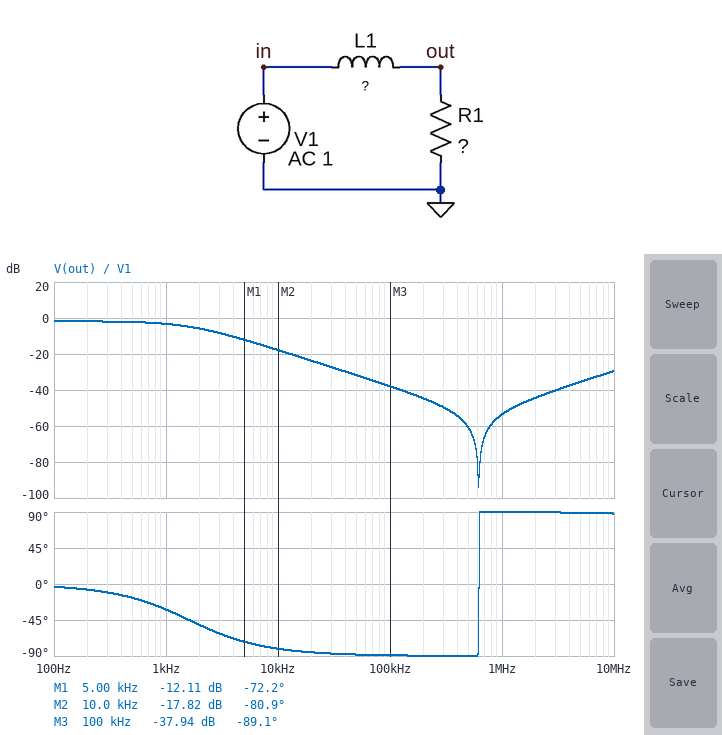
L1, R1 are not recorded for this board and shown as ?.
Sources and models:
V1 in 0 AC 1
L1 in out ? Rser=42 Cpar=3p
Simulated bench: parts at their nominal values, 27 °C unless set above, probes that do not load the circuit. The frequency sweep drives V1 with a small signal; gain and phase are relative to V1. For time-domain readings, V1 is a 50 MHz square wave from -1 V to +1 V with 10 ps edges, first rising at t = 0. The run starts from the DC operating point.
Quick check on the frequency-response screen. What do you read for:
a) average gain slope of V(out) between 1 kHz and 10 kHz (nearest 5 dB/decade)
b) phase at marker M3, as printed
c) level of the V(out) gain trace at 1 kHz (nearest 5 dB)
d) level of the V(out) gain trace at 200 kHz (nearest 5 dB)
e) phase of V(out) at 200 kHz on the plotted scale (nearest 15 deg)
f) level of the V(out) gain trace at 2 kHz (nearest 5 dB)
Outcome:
-15 dB/decade
-89.1 deg
-5 dB
-45 dB
-90 deg
-5 dB
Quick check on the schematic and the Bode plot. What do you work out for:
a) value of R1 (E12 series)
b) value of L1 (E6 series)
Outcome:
180 Ω
22 mH
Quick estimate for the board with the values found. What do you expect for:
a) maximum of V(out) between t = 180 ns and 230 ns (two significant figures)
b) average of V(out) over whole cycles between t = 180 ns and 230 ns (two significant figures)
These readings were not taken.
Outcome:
1.2 V
-810 mV
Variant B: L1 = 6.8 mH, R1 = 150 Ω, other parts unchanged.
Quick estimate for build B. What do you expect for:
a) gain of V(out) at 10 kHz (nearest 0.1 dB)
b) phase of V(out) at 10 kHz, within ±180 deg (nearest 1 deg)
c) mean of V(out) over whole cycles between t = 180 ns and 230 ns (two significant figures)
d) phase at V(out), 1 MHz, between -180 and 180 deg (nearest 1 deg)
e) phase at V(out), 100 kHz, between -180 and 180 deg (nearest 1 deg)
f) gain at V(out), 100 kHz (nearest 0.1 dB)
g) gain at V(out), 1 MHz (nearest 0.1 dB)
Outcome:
-9.9 dB
-66 deg
-780 mV
-90 deg
-87 deg
-29.2 dB
-63.3 dB
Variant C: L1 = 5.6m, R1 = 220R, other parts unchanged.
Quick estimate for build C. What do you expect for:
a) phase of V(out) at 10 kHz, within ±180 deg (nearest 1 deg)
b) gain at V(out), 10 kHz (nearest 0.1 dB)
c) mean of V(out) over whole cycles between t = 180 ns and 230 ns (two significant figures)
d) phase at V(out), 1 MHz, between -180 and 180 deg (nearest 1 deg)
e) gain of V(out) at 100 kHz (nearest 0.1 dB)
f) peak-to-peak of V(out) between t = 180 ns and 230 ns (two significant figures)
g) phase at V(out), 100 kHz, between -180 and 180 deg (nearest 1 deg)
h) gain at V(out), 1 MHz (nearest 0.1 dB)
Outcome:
-53 deg
-6.0 dB
-830 mV
-90 deg
-24.2 dB
4.0 V
-86 deg
-53.5 dB
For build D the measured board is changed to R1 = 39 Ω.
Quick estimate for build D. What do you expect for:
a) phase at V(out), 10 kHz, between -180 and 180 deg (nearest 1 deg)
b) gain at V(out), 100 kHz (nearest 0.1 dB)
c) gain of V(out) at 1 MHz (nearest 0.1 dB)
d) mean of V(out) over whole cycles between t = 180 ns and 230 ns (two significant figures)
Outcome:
-87 deg
-51.2 dB
-66.9 dB
-480 mV
